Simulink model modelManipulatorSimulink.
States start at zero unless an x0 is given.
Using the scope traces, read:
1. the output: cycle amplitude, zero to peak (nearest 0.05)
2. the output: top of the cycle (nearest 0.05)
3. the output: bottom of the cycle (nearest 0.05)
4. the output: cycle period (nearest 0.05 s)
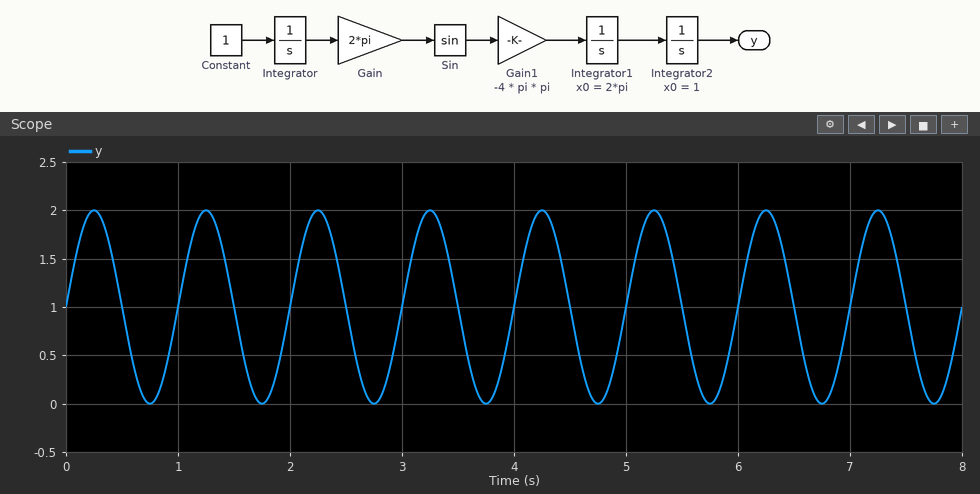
1.00
2.00
0.00
1.00 s
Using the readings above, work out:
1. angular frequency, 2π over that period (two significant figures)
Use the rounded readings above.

6.3 rad/s
